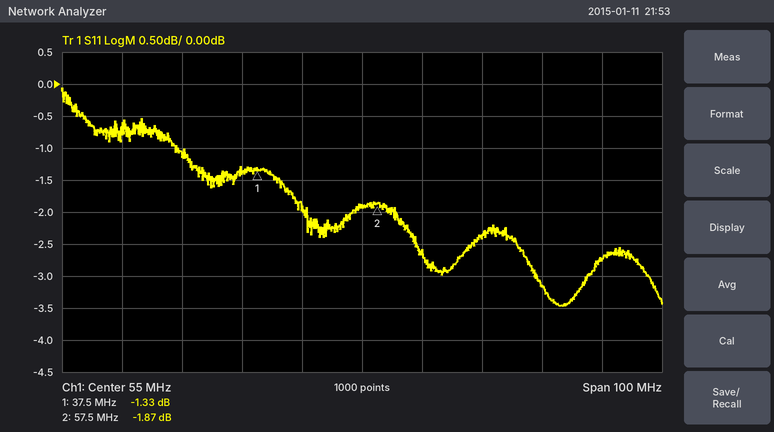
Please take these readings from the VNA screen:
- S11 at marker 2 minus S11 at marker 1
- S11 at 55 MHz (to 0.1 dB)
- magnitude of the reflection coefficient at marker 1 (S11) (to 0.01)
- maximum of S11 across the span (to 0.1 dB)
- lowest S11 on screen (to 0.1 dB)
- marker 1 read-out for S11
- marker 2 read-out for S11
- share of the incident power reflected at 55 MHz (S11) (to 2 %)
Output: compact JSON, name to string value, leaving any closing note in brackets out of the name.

{"S11 at marker 2 minus S11 at marker 1": "-0.54 dB", "S11 at 55 MHz": "-1.9 dB", "magnitude of the reflection coefficient at marker 1 (S11)": "0.86", "maximum of S11 across the span": "-0.1 dB", "lowest S11 on screen": "-3.5 dB", "marker 1 read-out for S11": "-1.33 dB", "marker 2 read-out for S11": "-1.87 dB", "share of the incident power reflected at 55 MHz (S11)": "64 %"}
